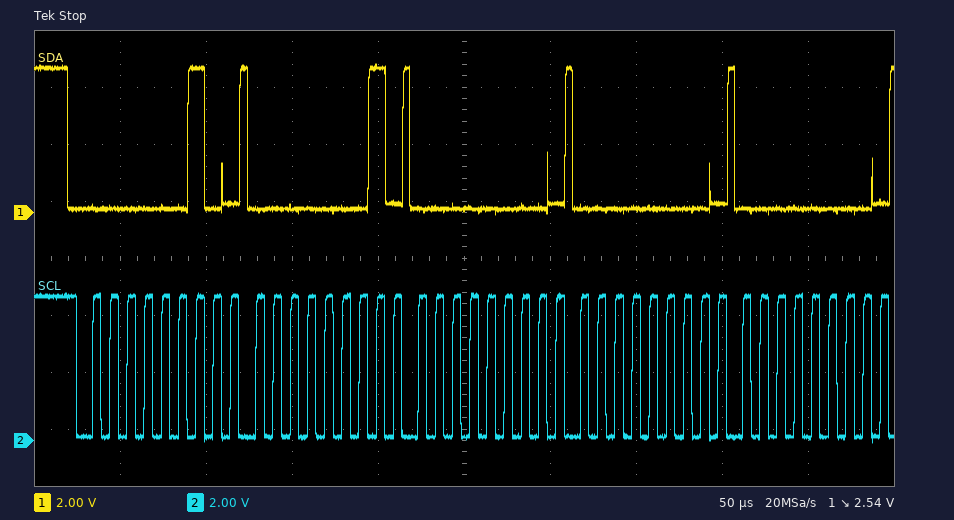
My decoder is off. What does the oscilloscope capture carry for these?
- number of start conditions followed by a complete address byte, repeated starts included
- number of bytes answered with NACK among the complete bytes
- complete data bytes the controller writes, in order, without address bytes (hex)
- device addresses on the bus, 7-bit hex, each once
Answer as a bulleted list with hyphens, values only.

- 1
- 0
- 01 00 00 00
- 0x01
